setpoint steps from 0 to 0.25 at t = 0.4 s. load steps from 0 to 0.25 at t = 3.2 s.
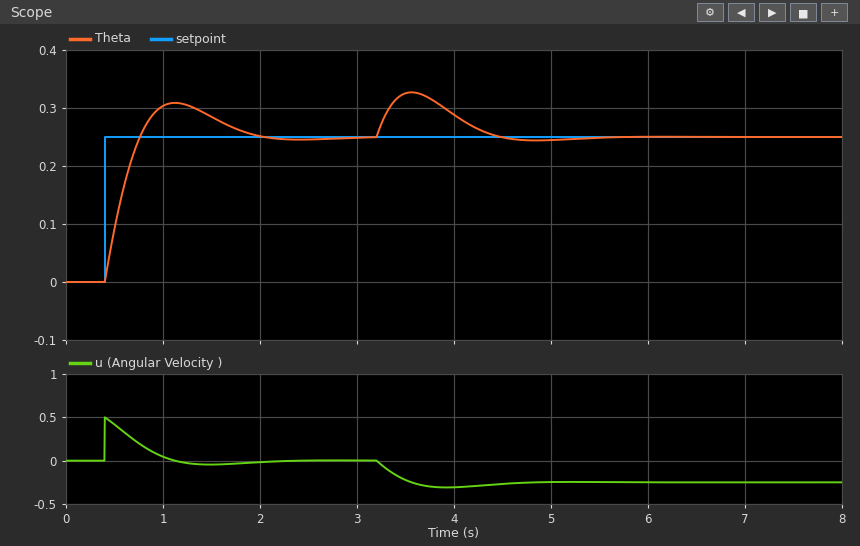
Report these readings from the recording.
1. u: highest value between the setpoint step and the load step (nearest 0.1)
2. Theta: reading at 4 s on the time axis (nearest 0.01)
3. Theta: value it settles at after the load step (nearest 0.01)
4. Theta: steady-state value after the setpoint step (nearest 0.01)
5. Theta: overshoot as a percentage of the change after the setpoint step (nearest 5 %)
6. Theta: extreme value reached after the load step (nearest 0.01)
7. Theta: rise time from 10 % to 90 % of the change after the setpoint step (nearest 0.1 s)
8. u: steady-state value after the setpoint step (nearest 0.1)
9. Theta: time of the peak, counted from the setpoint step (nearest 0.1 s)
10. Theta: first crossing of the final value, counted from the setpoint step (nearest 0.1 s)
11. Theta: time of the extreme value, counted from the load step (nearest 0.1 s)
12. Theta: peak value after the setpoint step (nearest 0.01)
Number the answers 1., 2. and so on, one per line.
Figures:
1. 0.5
2. 0.29
3. 0.25
4. 0.25
5. 25 %
6. 0.33
7. 0.3 s
8. 0.0
9. 0.7 s
10. 0.4 s
11. 0.4 s
12. 0.31
